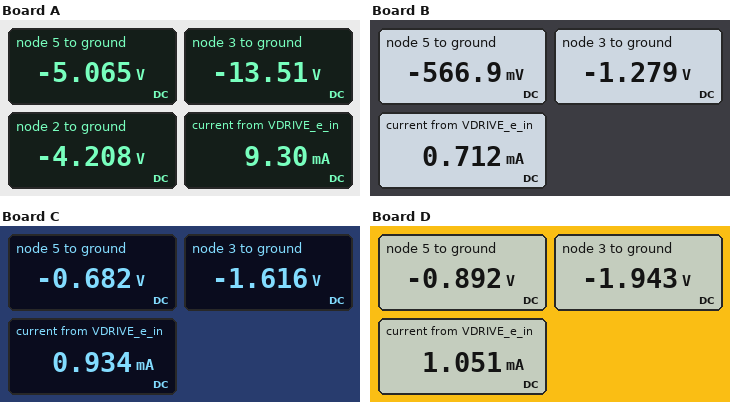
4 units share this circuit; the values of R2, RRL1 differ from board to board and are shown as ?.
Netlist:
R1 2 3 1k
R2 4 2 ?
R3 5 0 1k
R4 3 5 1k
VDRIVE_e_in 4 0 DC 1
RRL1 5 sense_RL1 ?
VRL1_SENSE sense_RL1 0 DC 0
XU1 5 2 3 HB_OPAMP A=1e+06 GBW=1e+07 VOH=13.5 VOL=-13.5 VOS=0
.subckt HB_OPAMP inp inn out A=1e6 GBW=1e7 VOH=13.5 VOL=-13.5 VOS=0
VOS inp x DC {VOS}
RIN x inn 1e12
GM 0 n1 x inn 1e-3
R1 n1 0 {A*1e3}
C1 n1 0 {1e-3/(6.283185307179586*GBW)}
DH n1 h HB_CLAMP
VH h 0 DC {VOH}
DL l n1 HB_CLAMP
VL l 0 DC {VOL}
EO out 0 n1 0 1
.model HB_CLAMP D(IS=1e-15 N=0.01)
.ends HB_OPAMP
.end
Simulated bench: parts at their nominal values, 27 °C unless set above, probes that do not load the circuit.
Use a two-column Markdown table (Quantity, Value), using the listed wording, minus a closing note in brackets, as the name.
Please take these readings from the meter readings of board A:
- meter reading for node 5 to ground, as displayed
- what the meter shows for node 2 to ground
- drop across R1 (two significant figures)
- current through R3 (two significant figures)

| Quantity | Value |
|---|---|
| meter reading for node 5 to ground, as displayed | -5.065 V |
| what the meter shows for node 2 to ground | -4.208 V |
| drop across R1 | 9.3 V |
| current through R3 | 5.1 mA |
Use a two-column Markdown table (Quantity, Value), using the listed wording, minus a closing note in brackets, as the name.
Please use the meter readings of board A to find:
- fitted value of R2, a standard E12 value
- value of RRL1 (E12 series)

| Quantity | Value |
|---|---|
| fitted value of R2, a standard E12 value | 560 Ω |
| value of RRL1 | 1.5 kΩ |
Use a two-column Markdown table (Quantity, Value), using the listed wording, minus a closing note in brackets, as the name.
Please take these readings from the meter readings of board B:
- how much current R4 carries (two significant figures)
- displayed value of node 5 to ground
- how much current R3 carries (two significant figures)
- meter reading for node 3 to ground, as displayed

| Quantity | Value |
|---|---|
| how much current R4 carries | 710 µA |
| displayed value of node 5 to ground | -566.9 mV |
| how much current R3 carries | 570 µA |
| meter reading for node 3 to ground, as displayed | -1.279 V |
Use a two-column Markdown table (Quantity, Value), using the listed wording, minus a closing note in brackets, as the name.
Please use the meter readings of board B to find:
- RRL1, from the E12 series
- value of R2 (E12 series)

| Quantity | Value |
|---|---|
| RRL1, from the E12 series | 3.9 kΩ |
| value of R2 | 2.2 kΩ |
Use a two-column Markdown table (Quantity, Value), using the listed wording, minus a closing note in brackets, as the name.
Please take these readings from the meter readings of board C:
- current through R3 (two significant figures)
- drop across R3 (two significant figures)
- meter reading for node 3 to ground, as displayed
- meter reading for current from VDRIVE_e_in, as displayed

| Quantity | Value |
|---|---|
| current through R3 | 680 µA |
| drop across R3 | 680 mV |
| meter reading for node 3 to ground, as displayed | -1.616 V |
| meter reading for current from VDRIVE_e_in, as displayed | 0.934 mA |
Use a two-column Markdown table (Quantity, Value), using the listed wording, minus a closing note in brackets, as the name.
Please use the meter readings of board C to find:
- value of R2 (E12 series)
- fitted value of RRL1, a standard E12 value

| Quantity | Value |
|---|---|
| value of R2 | 1.8 kΩ |
| fitted value of RRL1, a standard E12 value | 2.7 kΩ |
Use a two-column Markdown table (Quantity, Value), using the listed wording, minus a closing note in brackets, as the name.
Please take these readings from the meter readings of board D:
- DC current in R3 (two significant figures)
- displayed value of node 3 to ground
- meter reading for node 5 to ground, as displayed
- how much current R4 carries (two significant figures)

| Quantity | Value |
|---|---|
| DC current in R3 | 890 µA |
| displayed value of node 3 to ground | -1.943 V |
| meter reading for node 5 to ground, as displayed | -0.892 V |
| how much current R4 carries | 1.1 mA |
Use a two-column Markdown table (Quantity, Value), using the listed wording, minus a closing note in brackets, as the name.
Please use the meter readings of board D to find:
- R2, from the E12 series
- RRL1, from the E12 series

| Quantity | Value |
|---|---|
| R2, from the E12 series | 1.8 kΩ |
| RRL1, from the E12 series | 5.6 kΩ |
